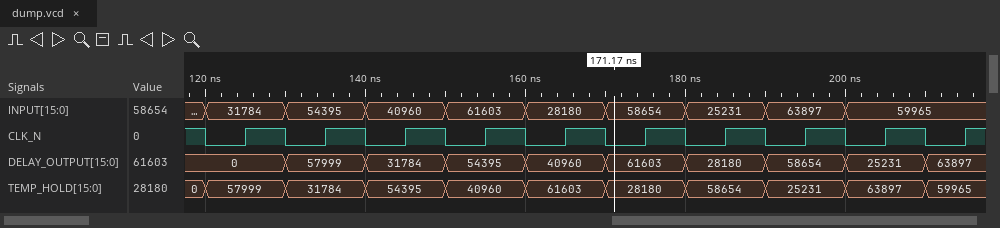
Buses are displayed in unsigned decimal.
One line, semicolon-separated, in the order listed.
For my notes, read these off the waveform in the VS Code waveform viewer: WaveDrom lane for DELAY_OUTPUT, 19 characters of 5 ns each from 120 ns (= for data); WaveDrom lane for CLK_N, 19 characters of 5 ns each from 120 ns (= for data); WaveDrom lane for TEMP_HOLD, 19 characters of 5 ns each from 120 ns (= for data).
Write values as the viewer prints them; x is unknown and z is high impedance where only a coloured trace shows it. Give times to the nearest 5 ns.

{name: 'DELAY_OUTPUT', wave: '=.=.=.=.=.=.=.=.=.=', data: '0 57999 31784 54395 40960 61603 28180 58654 25231 63897'}; {name: 'CLK_N', wave: '0101010101010101010'}; {name: 'TEMP_HOLD', wave: '=.=.=.=.=.=.=.=.=.=', data: '57999 31784 54395 40960 61603 28180 58654 25231 63897 59965'}
